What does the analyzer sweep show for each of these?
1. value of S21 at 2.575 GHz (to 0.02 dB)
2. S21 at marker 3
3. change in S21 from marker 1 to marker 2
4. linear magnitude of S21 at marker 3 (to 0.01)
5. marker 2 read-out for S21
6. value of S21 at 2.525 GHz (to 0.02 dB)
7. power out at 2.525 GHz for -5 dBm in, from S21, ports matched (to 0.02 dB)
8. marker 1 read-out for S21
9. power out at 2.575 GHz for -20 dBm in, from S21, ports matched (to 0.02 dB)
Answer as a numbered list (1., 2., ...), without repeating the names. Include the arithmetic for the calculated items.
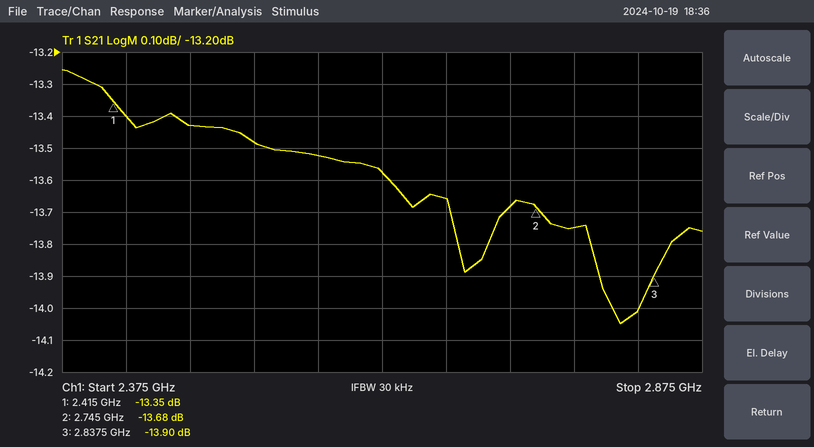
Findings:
1. -13.52 dB
2. -13.90 dB
3. -13.68 − (-13.35) = -0.33 dB
4. 10^(-13.9/20) ≈ 0.20
5. -13.68 dB
6. -13.48 dB
7. -5 dBm + (-13.48 dB) = -18.48 dBm
8. -13.35 dB
9. -20 dBm + (-13.52 dB) = -33.52 dBm
